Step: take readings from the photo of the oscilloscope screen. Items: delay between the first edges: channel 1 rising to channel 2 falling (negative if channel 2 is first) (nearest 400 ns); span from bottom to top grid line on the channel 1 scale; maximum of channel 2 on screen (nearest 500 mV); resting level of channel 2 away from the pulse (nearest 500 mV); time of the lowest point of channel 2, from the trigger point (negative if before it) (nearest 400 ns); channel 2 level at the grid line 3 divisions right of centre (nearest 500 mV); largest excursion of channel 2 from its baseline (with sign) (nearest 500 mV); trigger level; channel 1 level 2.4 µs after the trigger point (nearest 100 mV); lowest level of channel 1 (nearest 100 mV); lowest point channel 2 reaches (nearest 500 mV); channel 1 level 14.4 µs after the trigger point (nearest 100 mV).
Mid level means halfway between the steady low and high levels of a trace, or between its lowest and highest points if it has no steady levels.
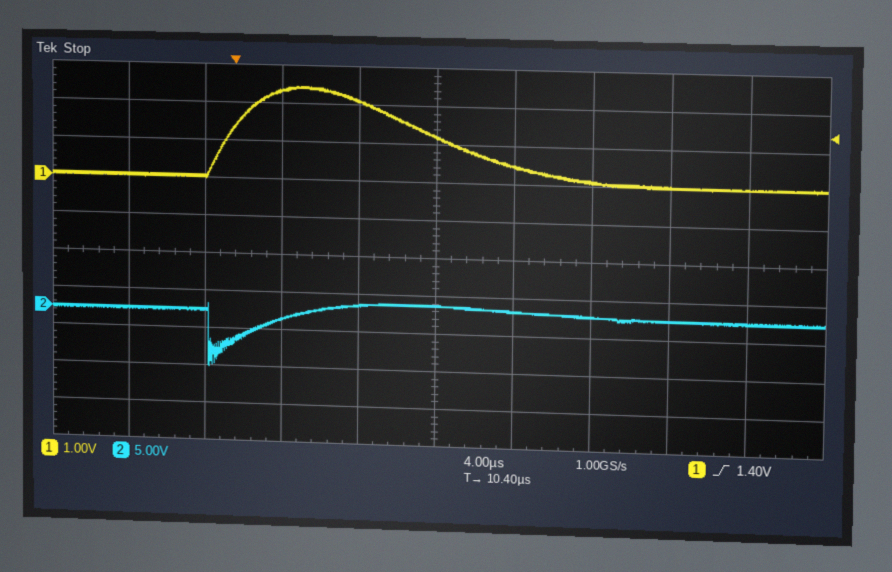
-1.2 µs
10 V
1.5 V
0.0 V
-1.2 µs
0.0 V
-7.5 V
1.40 V
2.3 V
0.0 V
-7.5 V
500 mV
